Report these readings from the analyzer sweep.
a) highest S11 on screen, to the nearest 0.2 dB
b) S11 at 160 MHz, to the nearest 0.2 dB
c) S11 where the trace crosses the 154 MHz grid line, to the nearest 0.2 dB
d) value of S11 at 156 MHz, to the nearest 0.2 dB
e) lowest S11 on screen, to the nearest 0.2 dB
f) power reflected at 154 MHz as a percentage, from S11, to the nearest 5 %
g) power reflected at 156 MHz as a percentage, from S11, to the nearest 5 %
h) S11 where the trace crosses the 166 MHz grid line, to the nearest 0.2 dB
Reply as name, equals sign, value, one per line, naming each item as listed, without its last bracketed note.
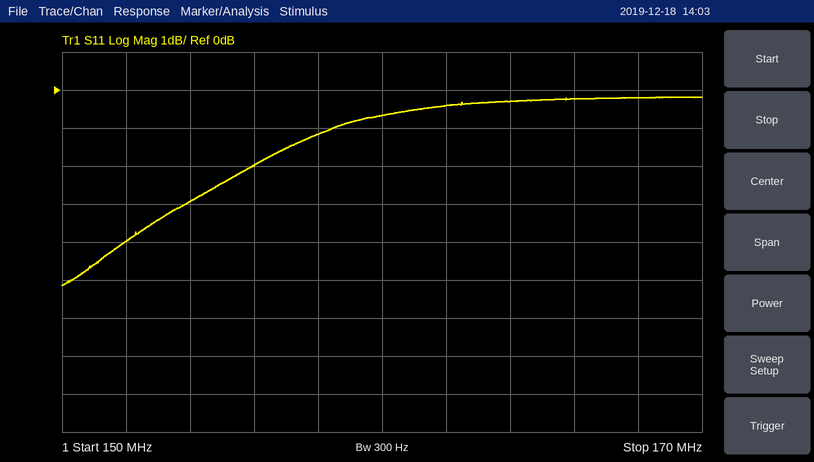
highest S11 on screen, to the nearest 0.2 dB = -0.2 dB
S11 at 160 MHz, to the nearest 0.2 dB = -0.6 dB
S11 where the trace crosses the 154 MHz grid line, to the nearest 0.2 dB = -3.0 dB
value of S11 at 156 MHz, to the nearest 0.2 dB = -2.0 dB
lowest S11 on screen, to the nearest 0.2 dB = -5.2 dB
power reflected at 154 MHz as a percentage, from S11, to the nearest 5 % = 50 %
power reflected at 156 MHz as a percentage, from S11, to the nearest 5 % = 65 %
S11 where the trace crosses the 166 MHz grid line, to the nearest 0.2 dB = -0.2 dB
